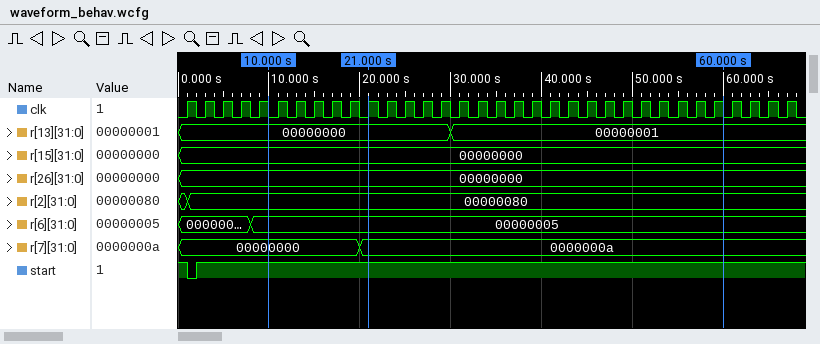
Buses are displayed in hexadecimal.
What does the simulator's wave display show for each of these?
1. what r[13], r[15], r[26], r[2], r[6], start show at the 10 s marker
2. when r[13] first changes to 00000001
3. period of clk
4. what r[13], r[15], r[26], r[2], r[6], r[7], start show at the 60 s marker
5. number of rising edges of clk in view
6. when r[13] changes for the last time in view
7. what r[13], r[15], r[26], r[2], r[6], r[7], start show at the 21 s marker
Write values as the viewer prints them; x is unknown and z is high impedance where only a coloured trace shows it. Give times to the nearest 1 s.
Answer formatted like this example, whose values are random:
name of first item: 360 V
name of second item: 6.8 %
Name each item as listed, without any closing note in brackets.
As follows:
what r[13], r[15], r[26], r[2], r[6], start show at the 10 s marker: r[13]=00000000, r[15]=00000000, r[26]=00000000, r[2]=00000080, r[6]=00000005, start=1
when r[13] first changes to 00000001: 30 s
period of clk: 2 s
what r[13], r[15], r[26], r[2], r[6], r[7], start show at the 60 s marker: r[13]=00000001, r[15]=00000000, r[26]=00000000, r[2]=00000080, r[6]=00000005, r[7]=0000000a, start=1
number of rising edges of clk in view: 34
when r[13] changes for the last time in view: 30 s
what r[13], r[15], r[26], r[2], r[6], r[7], start show at the 21 s marker: r[13]=00000000, r[15]=00000000, r[26]=00000000, r[2]=00000080, r[6]=00000005, r[7]=0000000a, start=1
